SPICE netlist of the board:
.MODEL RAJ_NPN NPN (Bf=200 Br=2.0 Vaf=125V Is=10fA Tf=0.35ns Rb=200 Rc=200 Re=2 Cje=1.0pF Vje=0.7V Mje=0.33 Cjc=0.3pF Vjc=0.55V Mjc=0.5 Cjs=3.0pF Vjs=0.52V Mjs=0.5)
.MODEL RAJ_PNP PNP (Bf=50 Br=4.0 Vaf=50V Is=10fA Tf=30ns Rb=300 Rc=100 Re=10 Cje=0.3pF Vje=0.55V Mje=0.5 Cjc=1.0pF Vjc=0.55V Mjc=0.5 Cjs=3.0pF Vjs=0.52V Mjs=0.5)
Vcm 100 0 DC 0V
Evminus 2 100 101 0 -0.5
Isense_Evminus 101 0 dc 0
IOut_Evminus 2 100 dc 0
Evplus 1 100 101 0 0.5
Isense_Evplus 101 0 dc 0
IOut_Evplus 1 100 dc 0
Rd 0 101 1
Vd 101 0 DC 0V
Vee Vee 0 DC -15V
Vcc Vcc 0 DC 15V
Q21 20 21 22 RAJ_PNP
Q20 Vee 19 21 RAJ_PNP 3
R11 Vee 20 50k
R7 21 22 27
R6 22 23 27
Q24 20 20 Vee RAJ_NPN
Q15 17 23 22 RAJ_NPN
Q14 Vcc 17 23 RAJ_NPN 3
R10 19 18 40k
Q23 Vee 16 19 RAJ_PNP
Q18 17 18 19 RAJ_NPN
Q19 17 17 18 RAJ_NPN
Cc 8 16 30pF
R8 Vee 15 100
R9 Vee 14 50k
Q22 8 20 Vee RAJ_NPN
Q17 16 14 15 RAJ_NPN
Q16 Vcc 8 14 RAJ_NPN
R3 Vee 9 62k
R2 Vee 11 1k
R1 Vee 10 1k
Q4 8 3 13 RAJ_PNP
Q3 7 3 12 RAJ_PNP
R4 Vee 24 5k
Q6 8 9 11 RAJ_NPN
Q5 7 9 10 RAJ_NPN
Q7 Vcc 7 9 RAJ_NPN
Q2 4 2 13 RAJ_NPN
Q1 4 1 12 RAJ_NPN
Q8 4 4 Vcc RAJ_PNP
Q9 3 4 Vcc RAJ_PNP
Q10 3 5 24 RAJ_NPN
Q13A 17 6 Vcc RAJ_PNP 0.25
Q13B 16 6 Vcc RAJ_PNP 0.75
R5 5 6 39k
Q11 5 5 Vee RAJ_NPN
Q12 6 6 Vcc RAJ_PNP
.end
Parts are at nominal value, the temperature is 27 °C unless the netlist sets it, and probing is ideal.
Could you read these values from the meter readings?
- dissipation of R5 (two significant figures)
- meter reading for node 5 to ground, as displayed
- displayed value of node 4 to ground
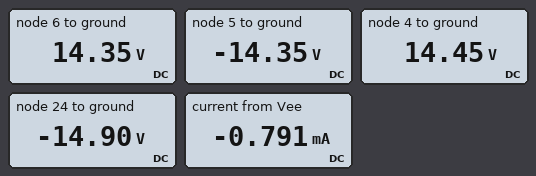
21 mW
-14.35 V
14.45 V
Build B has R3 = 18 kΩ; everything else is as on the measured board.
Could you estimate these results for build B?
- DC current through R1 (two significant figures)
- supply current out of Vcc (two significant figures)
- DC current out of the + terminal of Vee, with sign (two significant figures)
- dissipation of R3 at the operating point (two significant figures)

7.5 µA
2.0 mA
-2.0 mA
16 µW
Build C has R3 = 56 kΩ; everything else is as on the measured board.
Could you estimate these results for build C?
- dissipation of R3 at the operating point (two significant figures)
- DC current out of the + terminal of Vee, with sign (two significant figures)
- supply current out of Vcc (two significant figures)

5.1 µW
-800 µA
800 µA
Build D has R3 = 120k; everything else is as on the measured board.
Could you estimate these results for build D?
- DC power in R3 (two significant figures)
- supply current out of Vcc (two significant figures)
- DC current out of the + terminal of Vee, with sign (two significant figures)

2.4 µW
780 µA
-780 µA
